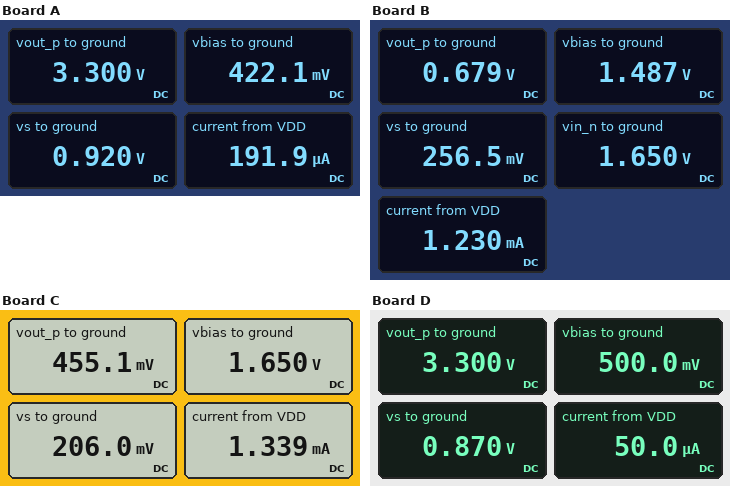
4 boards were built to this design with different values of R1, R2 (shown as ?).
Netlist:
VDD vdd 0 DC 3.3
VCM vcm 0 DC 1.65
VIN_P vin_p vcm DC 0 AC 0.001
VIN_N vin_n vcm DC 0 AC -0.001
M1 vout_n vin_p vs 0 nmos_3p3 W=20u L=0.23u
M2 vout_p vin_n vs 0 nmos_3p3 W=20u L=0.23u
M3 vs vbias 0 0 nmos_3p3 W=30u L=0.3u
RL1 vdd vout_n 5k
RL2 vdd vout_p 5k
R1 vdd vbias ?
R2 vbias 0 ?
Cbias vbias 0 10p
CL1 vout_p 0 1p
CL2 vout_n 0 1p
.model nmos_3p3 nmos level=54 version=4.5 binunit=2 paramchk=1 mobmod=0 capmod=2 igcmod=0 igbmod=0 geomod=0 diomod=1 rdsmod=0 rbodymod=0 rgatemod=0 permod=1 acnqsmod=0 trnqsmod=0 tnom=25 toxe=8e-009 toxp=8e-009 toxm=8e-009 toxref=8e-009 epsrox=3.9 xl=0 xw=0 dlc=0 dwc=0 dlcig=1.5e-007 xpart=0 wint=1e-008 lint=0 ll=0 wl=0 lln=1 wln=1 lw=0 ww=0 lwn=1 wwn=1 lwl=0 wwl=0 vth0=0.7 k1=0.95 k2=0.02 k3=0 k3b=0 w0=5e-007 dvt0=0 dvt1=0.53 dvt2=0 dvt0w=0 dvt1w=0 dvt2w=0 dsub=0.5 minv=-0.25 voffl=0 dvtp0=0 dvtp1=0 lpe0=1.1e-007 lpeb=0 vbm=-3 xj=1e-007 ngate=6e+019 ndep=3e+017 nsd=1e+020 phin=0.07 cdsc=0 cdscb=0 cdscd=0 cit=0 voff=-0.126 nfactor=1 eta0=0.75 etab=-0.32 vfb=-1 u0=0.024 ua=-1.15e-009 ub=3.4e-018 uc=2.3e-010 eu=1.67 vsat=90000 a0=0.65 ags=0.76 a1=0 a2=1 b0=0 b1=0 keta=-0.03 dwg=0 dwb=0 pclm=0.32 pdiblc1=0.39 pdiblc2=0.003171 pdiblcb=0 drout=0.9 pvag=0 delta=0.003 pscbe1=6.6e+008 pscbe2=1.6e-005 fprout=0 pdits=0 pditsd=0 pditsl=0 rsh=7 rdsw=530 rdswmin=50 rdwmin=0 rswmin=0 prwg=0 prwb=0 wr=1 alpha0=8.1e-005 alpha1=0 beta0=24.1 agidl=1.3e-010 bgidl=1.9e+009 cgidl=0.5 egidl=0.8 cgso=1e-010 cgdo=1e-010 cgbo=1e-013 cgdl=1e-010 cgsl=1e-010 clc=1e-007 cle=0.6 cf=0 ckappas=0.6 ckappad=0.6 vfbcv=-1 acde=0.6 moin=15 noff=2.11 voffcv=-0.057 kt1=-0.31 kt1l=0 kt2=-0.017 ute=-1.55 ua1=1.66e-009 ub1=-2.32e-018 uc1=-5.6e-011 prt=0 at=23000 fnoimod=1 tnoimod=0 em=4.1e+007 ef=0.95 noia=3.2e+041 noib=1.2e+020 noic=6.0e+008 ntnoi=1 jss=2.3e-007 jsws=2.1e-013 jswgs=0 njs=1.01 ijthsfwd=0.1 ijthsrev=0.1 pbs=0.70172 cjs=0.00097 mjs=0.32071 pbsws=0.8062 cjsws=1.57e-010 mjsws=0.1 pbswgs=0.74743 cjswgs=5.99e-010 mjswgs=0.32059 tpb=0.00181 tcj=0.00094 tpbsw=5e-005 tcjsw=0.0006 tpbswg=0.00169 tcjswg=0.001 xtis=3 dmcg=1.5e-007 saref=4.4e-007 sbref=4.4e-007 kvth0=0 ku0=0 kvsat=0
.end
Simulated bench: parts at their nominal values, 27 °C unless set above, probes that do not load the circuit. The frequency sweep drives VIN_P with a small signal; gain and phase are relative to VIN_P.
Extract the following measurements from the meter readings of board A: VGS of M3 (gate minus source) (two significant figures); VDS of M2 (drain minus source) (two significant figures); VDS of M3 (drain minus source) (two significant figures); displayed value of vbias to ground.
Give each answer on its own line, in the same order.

420 mV
2.4 V
920 mV
422.1 mV
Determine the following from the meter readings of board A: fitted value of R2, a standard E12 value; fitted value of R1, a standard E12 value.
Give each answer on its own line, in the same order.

2.2 kΩ
15 kΩ
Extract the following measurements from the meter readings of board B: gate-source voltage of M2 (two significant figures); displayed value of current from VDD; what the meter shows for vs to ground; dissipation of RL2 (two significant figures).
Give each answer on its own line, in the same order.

1.4 V
1.230 mA
256.5 mV
1.4 mW
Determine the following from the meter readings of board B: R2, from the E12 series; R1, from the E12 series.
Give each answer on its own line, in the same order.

8.2 kΩ
10 kΩ
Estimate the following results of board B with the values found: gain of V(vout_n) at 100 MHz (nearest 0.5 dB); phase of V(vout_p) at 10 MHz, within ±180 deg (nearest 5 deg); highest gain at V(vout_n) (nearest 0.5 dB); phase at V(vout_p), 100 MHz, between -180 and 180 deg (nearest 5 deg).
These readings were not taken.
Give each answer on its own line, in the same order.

5.0 dB
-5 deg
10.5 dB
-50 deg
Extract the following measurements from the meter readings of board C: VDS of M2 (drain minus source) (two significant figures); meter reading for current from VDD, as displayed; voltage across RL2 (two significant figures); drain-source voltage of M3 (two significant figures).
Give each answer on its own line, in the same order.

250 mV
1.339 mA
2.8 V
210 mV
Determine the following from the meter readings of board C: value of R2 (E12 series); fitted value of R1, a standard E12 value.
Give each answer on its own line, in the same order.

8.2 kΩ
8.2 kΩ
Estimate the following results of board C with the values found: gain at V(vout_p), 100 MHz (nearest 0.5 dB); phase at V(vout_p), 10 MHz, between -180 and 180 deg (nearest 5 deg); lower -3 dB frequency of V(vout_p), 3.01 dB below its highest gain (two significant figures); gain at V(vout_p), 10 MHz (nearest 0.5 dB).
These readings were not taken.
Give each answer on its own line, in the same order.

-12.5 dB
10 deg
47 MHz
-19.0 dB
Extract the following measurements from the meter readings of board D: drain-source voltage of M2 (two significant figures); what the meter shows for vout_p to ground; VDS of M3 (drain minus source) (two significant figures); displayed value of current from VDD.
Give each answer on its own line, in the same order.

2.4 V
3.300 V
870 mV
50.0 µA
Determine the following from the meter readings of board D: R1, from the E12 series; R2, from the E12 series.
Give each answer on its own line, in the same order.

56 kΩ
10 kΩ
